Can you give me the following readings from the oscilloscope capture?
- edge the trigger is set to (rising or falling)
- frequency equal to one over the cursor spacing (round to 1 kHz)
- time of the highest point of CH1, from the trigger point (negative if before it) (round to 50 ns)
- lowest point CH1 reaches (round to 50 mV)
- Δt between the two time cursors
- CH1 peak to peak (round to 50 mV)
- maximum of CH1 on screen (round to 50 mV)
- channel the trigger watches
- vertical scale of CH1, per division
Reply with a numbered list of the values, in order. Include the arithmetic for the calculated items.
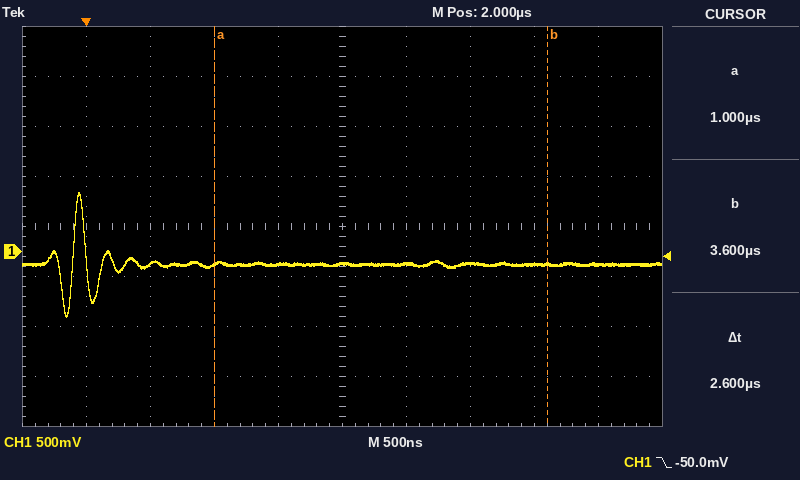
1. falling
2. 1 / 2.6 µs ≈ 385 kHz
3. -50 ns
4. -650 mV
5. 2.6 µs
6. 600 mV − (-650 mV) = 1.25 V
7. 600 mV
8. CH1
9. 500 mV
